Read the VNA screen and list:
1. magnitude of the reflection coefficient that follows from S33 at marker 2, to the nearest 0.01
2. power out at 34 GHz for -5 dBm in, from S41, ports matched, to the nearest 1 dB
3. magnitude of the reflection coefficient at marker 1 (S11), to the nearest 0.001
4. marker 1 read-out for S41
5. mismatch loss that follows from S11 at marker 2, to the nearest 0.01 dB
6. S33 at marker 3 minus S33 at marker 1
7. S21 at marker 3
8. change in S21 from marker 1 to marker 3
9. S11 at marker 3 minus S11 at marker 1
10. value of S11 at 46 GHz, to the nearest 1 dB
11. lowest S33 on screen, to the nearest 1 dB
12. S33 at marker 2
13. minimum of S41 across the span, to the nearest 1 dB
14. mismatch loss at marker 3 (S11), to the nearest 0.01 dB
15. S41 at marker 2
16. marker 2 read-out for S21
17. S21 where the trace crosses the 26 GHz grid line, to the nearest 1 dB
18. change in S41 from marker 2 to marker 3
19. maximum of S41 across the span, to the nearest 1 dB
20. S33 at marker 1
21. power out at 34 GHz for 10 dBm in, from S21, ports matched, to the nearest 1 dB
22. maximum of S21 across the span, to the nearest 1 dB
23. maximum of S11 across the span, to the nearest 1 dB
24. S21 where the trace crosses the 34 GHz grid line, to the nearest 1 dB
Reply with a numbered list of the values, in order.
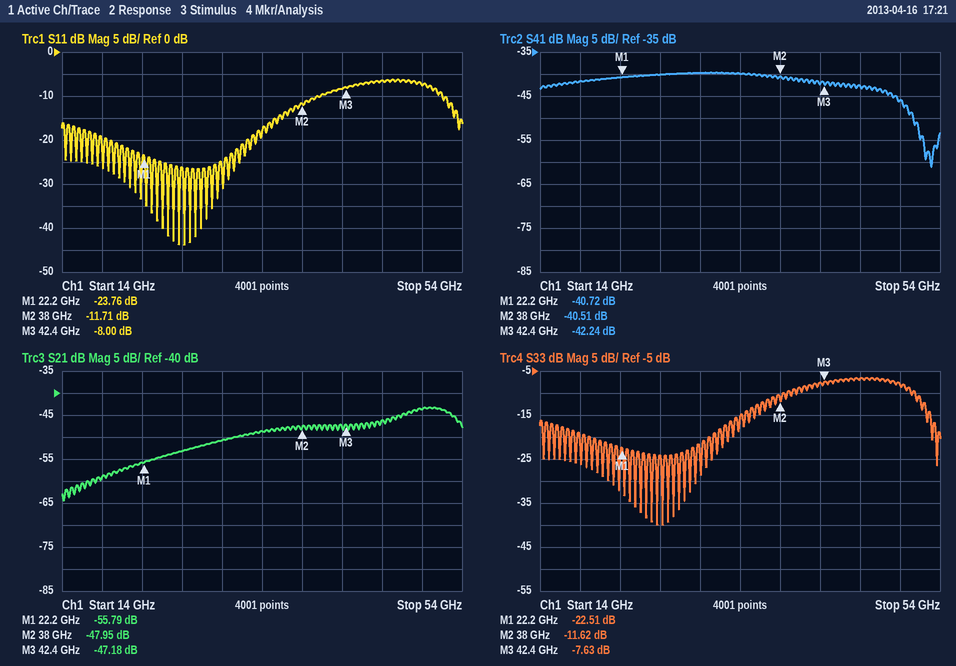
1. 0.26
2. -45 dBm
3. 0.065
4. -40.72 dB
5. 0.30 dB
6. 14.88 dB
7. -47.18 dB
8. 8.61 dB
9. 15.76 dB
10. -6 dB
11. -40 dB
12. -11.62 dB
13. -61 dB
14. 0.75 dB
15. -40.51 dB
16. -47.95 dB
17. -53 dB
18. -1.73 dB
19. -40 dB
20. -22.51 dB
21. -39 dBm
22. -43 dB
23. -6 dB
24. -49 dB
